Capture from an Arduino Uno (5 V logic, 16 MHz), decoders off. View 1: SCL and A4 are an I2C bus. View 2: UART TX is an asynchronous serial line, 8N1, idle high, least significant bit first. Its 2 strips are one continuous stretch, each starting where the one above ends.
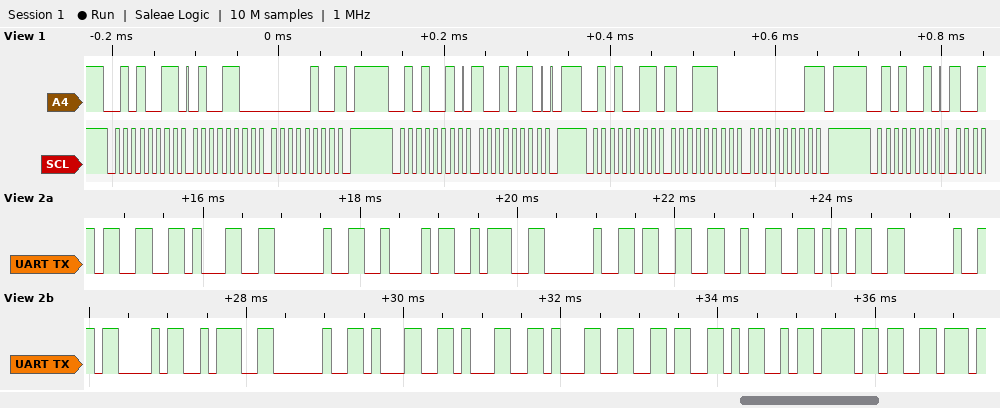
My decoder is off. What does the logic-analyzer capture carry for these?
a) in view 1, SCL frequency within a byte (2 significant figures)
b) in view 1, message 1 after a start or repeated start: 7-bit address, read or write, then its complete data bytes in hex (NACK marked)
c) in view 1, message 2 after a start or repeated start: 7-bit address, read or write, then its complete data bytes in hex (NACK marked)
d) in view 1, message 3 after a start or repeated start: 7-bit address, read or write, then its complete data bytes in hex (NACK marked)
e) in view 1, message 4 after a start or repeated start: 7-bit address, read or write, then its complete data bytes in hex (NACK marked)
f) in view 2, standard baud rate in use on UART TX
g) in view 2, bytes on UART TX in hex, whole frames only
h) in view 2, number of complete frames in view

100 kHz
0x29 read: 4C 04 NACK
0x29 write: 96
0x29 read: 9C 01 NACK
0x29 write
9600 baud
33 31 20 42 3A 20 33 32 35 20 43 3A 20 31 31 31 36 4D 6F 76
20
